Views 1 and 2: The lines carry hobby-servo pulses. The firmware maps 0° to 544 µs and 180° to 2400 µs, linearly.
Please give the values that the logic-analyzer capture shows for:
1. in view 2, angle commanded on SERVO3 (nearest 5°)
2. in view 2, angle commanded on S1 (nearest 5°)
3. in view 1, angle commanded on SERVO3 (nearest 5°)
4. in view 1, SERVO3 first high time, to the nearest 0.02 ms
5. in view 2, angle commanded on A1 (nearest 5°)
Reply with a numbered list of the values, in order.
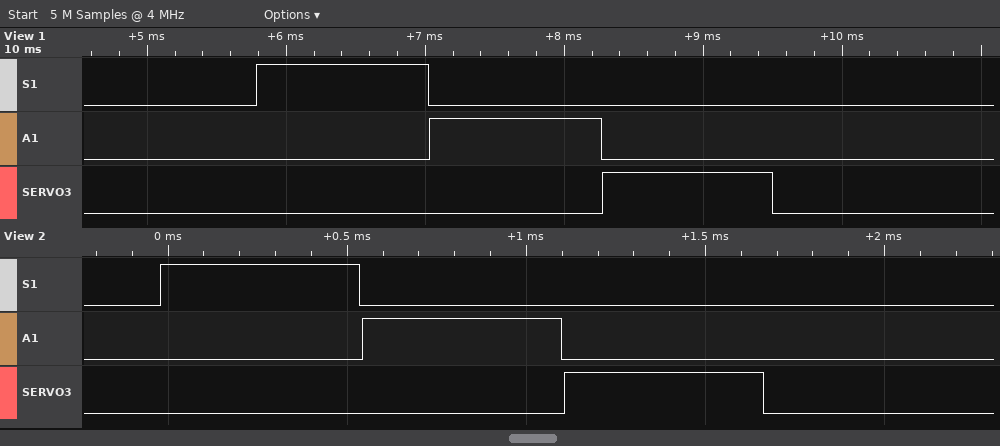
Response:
1. 0°
2. 0°
3. 65°
4. 1.22 ms
5. 0°
